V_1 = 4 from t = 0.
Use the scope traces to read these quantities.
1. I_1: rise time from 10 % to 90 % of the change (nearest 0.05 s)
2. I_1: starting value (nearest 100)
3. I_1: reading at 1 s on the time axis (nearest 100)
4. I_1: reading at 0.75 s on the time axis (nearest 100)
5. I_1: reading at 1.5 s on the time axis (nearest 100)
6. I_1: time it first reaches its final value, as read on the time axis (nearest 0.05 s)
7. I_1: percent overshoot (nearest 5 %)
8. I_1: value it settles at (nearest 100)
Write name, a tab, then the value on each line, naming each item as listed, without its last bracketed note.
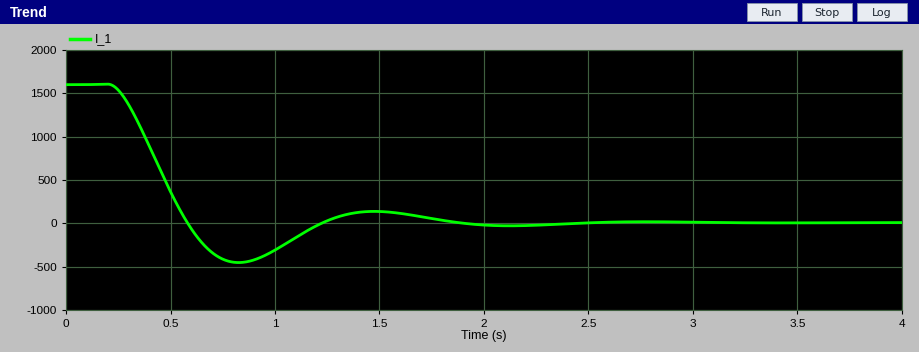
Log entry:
I_1: rise time from 10 % to 90 % of the change	0.25 s
I_1: starting value	1600
I_1: reading at 1 s on the time axis	-300
I_1: reading at 0.75 s on the time axis	-400
I_1: reading at 1.5 s on the time axis	100
I_1: time it first reaches its final value, as read on the time axis	0.60 s
I_1: percent overshoot	30 %
I_1: value it settles at	0
